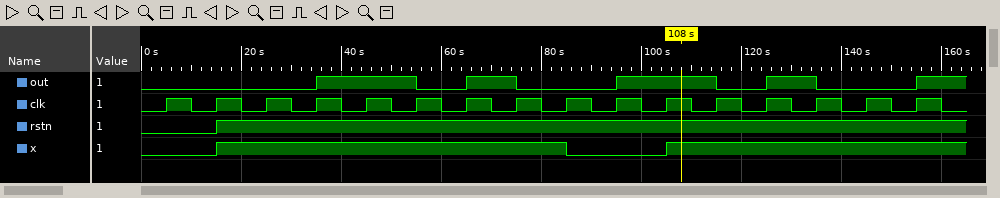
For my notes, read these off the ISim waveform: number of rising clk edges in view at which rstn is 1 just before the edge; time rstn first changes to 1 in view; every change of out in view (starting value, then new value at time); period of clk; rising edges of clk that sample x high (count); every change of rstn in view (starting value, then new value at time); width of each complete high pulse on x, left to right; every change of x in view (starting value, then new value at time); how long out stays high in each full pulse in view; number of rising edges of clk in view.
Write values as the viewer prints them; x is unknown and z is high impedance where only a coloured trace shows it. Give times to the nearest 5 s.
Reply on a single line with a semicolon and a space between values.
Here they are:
14; 15 s; 0, 1 at 35 s, 0 at 55 s, 1 at 65 s, 0 at 75 s, 1 at 95 s, 0 at 115 s, 1 at 125 s, 0 at 135 s, 1 at 155 s; 10 s; 12; 0, 1 at 15 s; 70 s; 0, 1 at 15 s, 0 at 85 s, 1 at 105 s; 20 s, 10 s, 20 s, 10 s; 16
